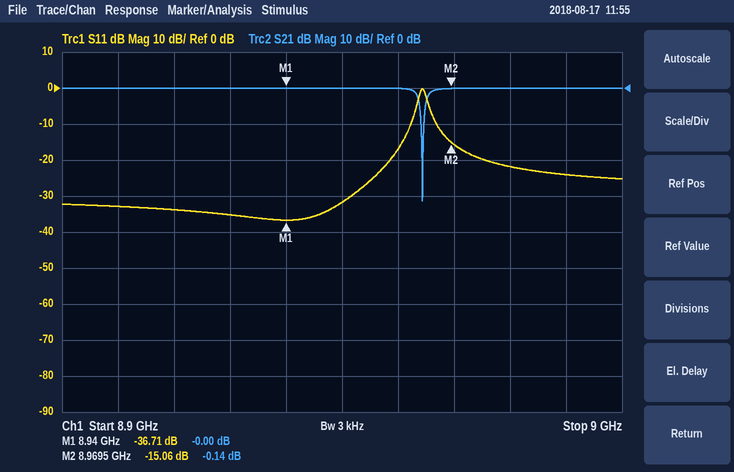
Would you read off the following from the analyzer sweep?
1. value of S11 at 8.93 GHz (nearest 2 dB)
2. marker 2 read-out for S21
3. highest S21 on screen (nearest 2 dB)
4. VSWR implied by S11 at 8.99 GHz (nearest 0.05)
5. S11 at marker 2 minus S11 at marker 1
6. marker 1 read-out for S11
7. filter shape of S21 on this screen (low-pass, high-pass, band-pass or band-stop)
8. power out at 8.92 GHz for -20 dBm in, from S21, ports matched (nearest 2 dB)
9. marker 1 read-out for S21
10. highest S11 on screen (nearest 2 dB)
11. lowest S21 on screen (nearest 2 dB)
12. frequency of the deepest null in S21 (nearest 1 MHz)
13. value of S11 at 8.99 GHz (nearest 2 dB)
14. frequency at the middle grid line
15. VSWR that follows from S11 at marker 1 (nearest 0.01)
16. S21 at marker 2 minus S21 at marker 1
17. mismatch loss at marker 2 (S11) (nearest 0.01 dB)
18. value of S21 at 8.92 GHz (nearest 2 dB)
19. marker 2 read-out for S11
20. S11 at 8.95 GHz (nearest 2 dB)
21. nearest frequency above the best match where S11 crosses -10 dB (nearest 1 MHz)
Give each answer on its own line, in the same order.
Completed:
-36 dB
-0.14 dB
0 dB
1.15
21.65 dB
-36.71 dB
band-stop
-20 dBm
-0.00 dB
0 dB
-32 dB
8.964 GHz
-24 dB
8.95 GHz
1.03
-0.14 dB
0.14 dB
0 dB
-15.06 dB
-32 dB
8.962 GHz
